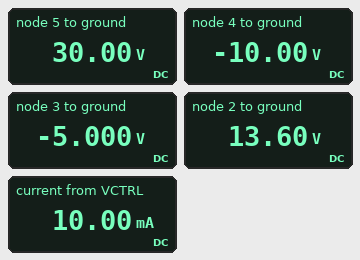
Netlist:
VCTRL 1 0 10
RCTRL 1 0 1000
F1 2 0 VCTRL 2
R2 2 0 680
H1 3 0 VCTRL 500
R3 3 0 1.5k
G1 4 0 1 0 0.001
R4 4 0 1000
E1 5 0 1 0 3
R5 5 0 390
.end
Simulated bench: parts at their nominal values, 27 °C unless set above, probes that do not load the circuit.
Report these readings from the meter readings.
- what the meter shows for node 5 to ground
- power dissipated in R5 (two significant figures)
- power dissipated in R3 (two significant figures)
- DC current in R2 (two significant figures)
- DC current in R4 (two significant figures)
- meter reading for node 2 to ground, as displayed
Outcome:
30.00 V
2.3 W
17 mW
20 mA
10 mA
13.60 V
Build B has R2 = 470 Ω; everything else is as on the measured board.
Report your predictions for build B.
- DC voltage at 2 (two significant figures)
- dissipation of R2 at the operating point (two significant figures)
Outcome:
9.4 V
190 mW
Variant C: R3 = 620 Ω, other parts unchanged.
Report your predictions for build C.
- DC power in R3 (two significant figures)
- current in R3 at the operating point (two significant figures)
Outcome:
40 mW
8.1 mA
